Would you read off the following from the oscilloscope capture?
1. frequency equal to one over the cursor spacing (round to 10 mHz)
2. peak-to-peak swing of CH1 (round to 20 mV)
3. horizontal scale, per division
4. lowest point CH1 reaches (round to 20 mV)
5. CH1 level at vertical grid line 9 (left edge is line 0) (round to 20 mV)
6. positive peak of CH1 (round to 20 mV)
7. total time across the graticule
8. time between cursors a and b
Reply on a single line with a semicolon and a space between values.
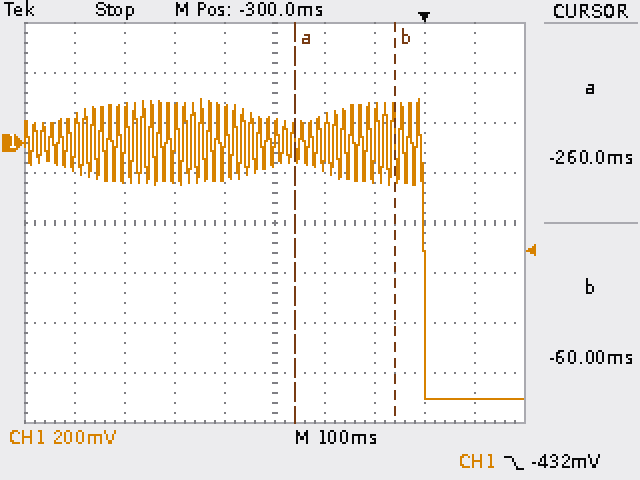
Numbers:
5.00 Hz; 1.20 V; 100 ms; -1.02 V; -1.02 V; 180 mV; 1 s; 200 ms
